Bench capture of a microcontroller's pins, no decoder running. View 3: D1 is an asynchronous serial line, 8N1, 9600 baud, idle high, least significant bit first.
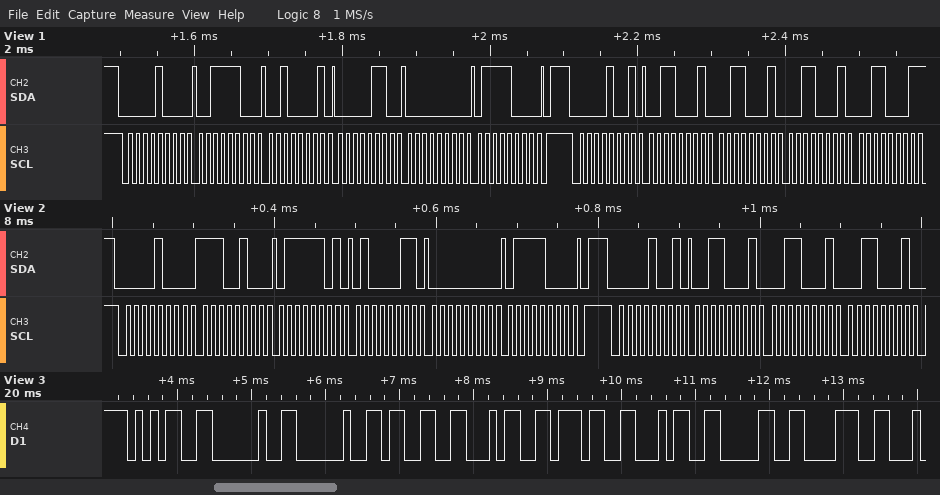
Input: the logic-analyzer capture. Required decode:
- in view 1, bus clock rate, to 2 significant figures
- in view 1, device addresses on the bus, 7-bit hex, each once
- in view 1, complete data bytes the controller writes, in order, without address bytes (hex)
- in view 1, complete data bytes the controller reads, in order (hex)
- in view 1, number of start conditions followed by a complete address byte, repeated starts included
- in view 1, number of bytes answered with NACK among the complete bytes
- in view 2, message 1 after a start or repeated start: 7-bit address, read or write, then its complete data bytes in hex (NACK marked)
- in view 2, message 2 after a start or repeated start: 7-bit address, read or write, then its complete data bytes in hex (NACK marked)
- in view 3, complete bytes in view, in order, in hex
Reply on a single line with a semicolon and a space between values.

100 kHz; 0x04; 3C 21 06 00 78; 31 31 31 31; 2; 1; 0x04 write: E4 7D 43 00 78; 0x04 read: 31 31 31; 35 20 20 33 34 37 34 30 38
